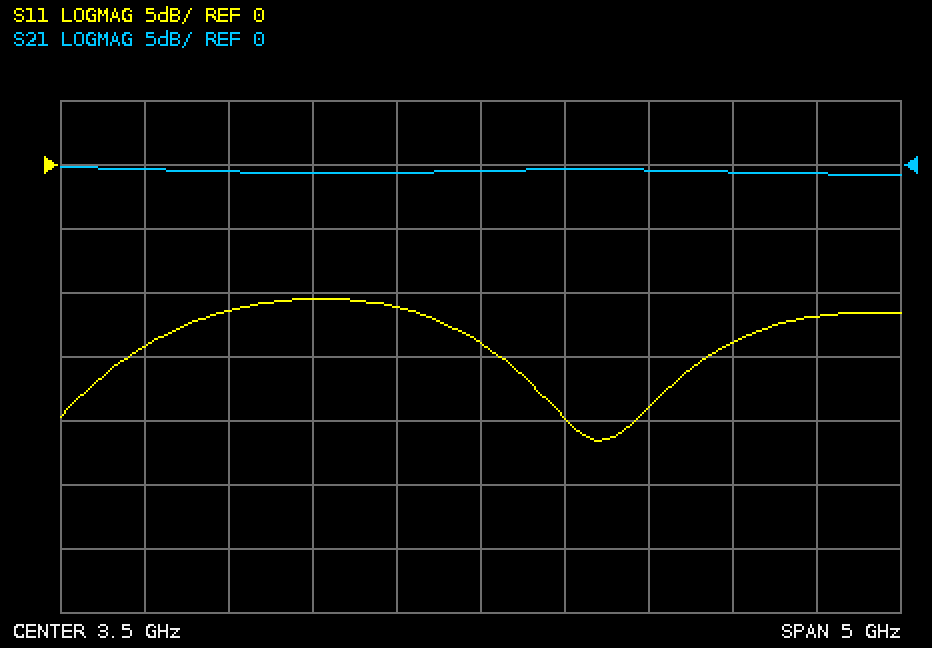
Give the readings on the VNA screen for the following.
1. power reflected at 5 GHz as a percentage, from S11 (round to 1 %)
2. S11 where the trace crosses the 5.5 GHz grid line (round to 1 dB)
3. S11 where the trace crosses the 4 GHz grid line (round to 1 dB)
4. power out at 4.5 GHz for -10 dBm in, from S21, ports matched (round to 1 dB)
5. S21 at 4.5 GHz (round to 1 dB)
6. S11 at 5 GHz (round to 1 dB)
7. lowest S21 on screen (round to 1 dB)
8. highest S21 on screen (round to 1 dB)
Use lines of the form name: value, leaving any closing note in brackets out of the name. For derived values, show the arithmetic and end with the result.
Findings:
power reflected at 5 GHz as a percentage, from S11: 10^(-14/10) ≈ 4 %
S11 where the trace crosses the 5.5 GHz grid line: -12 dB
S11 where the trace crosses the 4 GHz grid line: -20 dB
power out at 4.5 GHz for -10 dBm in, from S21, ports matched: -10 dBm + (0 dB) = -10 dBm
S21 at 4.5 GHz: 0 dB
S11 at 5 GHz: -14 dB
lowest S21 on screen: -1 dB
highest S21 on screen: 0 dB
